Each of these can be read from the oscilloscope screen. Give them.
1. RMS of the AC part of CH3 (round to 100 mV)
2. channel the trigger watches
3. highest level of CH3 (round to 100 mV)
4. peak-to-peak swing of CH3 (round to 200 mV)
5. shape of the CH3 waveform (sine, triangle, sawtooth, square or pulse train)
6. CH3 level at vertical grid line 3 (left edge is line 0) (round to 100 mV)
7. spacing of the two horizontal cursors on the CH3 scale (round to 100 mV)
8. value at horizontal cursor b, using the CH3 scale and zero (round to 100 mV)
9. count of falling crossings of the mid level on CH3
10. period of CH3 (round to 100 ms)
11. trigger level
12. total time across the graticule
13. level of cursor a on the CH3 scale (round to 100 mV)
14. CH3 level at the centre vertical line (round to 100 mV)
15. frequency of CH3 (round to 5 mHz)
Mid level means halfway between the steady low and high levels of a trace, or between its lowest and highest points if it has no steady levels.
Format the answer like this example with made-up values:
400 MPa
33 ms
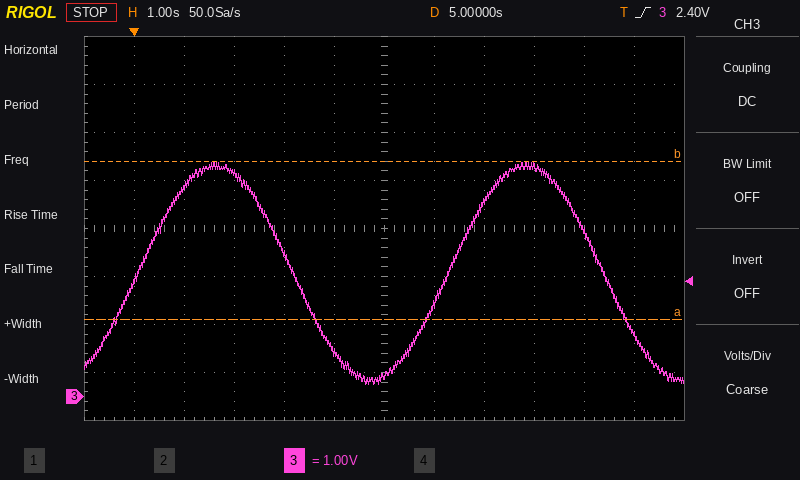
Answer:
1.6 V
CH3
4.9 V
4.6 V
sine
4.6 V
3.3 V
4.9 V
2
6.2 s
2.40 V
12 s
1.6 V
400 mV
160 mHz
